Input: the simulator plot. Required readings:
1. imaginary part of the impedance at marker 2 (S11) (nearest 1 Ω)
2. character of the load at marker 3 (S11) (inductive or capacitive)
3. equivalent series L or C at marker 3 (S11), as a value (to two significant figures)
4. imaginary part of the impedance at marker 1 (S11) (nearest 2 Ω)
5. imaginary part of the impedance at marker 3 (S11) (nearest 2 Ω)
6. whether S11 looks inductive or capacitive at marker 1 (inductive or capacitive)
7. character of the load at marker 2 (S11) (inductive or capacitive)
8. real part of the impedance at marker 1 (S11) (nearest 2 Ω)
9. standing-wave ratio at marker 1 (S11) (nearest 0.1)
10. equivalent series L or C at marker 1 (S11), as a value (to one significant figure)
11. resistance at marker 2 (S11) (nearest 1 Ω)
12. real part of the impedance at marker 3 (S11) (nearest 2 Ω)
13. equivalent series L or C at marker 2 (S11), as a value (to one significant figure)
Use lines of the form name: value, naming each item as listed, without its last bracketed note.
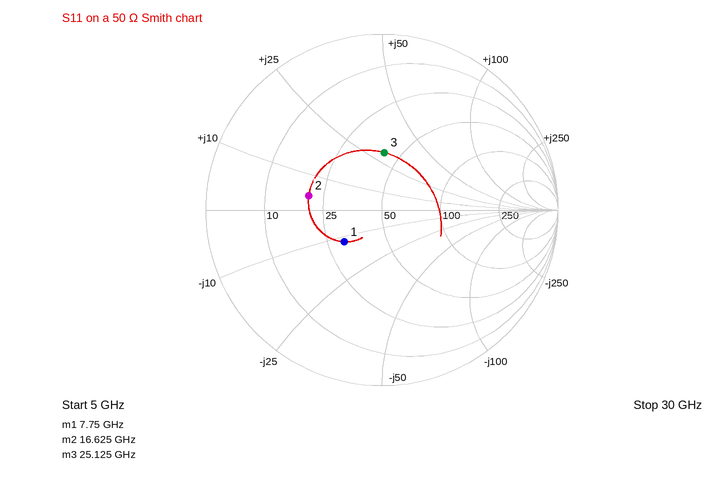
imaginary part of the impedance at marker 2 (S11): +4 Ω
character of the load at marker 3 (S11): inductive
equivalent series L or C at marker 3 (S11), as a value: 190 pH
imaginary part of the impedance at marker 1 (S11): -12 Ω
imaginary part of the impedance at marker 3 (S11): +30 Ω
whether S11 looks inductive or capacitive at marker 1: capacitive
character of the load at marker 2 (S11): inductive
real part of the impedance at marker 1 (S11): 30 Ω
standing-wave ratio at marker 1 (S11): 1.8
equivalent series L or C at marker 1 (S11), as a value: 2 pF
resistance at marker 2 (S11): 20 Ω
real part of the impedance at marker 3 (S11): 42 Ω
equivalent series L or C at marker 2 (S11), as a value: 40 pH
